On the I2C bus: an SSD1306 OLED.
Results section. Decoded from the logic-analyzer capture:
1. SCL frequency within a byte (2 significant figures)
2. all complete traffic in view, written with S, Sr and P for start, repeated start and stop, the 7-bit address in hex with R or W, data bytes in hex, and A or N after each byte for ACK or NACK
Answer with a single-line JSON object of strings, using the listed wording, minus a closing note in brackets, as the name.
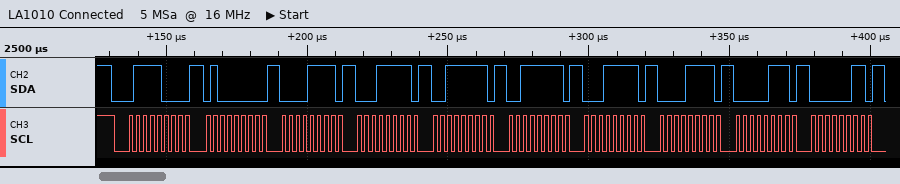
{"SCL frequency within a byte": "400 kHz", "all complete traffic in view, written with S, Sr and P for start, repeated start and stop, the 7-bit address in hex with R or W, data bytes in hex, and A or N after each byte for ACK or NACK": "S 3CW A 40 A 0F A 1F A 3F A 3F A 1F A 0F A 07 A 03 A"}
